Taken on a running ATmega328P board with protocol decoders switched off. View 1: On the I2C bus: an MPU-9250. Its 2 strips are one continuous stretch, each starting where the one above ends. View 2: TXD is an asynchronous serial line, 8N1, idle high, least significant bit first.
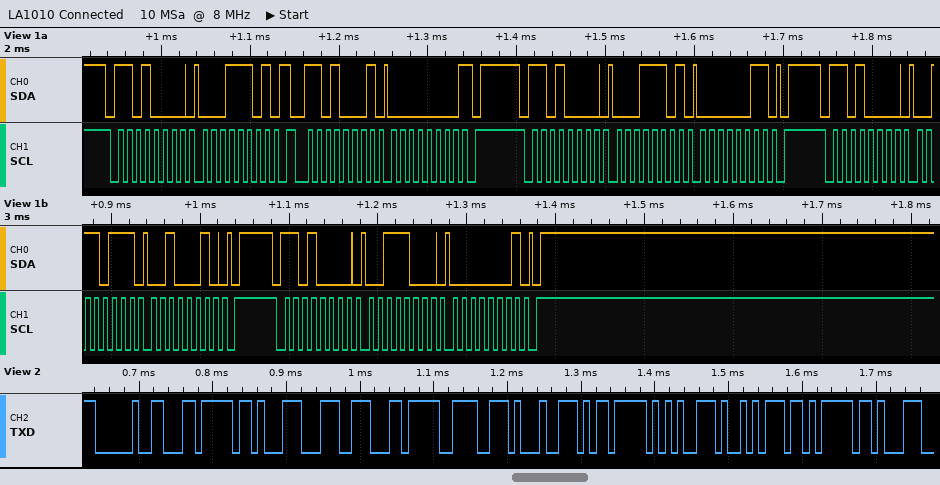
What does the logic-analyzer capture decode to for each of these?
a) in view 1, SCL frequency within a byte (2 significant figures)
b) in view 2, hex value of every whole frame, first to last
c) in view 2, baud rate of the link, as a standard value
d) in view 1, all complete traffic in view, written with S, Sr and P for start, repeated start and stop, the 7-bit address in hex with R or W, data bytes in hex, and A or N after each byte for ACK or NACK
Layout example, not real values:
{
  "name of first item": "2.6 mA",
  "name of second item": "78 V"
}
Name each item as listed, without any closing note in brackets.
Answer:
{
  "in view 1, SCL frequency within a byte": "100 kHz",
  "in view 2, hex value of every whole frame, first to last": "20 EC 8B 9C EC 9E 91 ED 95 A9 EB 8B",
  "in view 2, baud rate of the link, as a standard value": "115200 baud",
  "in view 1, all complete traffic in view, written with S, Sr and P for start, repeated start and stop, the 7-bit address in hex with R or W, data bytes in hex, and A or N after each byte for ACK or NACK": "S 68W A 1D A Sr 68R A 00 N P S 68W A 1D A 03 A P S 68W A 37 A 22 A P S 68W A 38 A 01 A P"
}
